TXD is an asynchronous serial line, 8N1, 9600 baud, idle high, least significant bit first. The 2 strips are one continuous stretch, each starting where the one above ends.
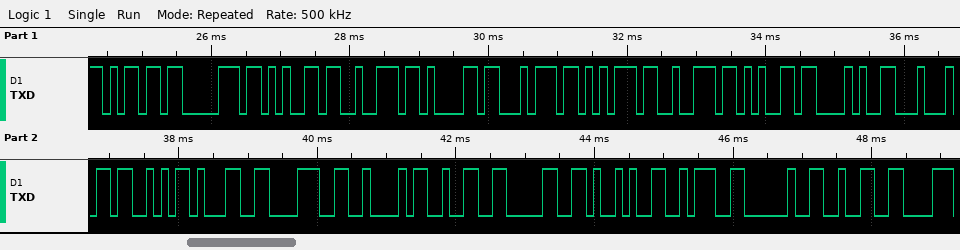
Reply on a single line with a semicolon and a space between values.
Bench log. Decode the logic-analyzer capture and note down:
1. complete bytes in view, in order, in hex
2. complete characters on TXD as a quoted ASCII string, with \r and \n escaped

6D 70 65 72 61 74 75 72 65 28 44 53 31 38 42 32 30 29 3A 20 32; "mperature(DS18B20): 2"
